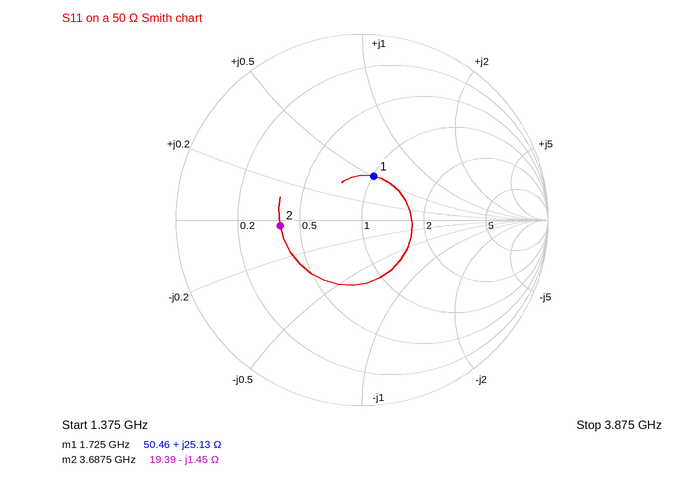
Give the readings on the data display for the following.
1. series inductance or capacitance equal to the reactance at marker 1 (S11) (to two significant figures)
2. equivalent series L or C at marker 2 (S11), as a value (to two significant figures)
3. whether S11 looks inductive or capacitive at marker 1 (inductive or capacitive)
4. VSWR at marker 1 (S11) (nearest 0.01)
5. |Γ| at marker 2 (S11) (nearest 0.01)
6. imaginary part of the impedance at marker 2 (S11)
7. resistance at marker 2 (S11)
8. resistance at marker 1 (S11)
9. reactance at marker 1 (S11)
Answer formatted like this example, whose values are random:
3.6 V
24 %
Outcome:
2.3 nH
30 pF
inductive
1.64
0.44
-1.45 Ω
19.39 Ω
50.46 Ω
+25.13 Ω
